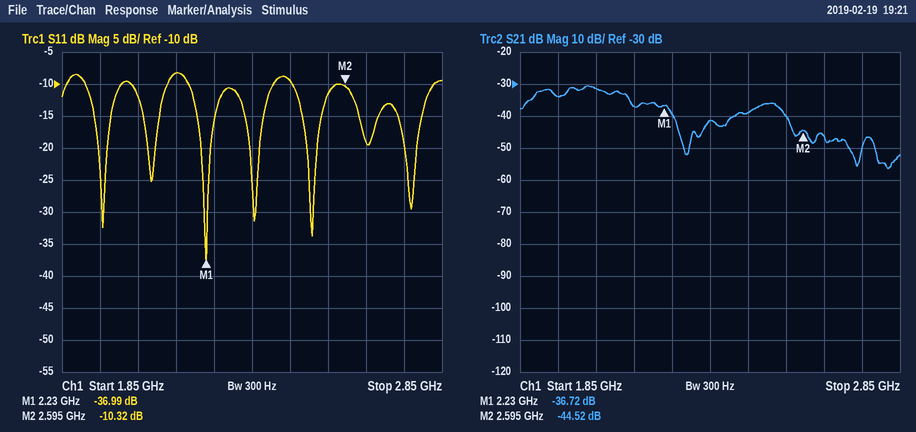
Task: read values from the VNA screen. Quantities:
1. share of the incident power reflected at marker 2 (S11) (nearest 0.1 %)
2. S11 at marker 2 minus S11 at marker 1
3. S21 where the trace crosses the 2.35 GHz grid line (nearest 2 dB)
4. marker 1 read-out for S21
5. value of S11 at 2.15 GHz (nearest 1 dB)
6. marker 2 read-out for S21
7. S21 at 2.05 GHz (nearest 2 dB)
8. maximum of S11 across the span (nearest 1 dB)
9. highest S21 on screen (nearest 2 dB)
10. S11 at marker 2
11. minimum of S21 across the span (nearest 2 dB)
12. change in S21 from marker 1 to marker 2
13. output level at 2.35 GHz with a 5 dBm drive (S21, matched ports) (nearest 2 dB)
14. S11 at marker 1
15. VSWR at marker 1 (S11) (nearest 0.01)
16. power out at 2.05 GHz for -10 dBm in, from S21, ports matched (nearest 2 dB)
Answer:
9.3 %
26.67 dB
-42 dB
-36.72 dB
-8 dB
-44.52 dB
-32 dB
-8 dB
-30 dB
-10.32 dB
-56 dB
-7.80 dB
-36 dBm
-36.99 dB
1.03
-42 dBm
